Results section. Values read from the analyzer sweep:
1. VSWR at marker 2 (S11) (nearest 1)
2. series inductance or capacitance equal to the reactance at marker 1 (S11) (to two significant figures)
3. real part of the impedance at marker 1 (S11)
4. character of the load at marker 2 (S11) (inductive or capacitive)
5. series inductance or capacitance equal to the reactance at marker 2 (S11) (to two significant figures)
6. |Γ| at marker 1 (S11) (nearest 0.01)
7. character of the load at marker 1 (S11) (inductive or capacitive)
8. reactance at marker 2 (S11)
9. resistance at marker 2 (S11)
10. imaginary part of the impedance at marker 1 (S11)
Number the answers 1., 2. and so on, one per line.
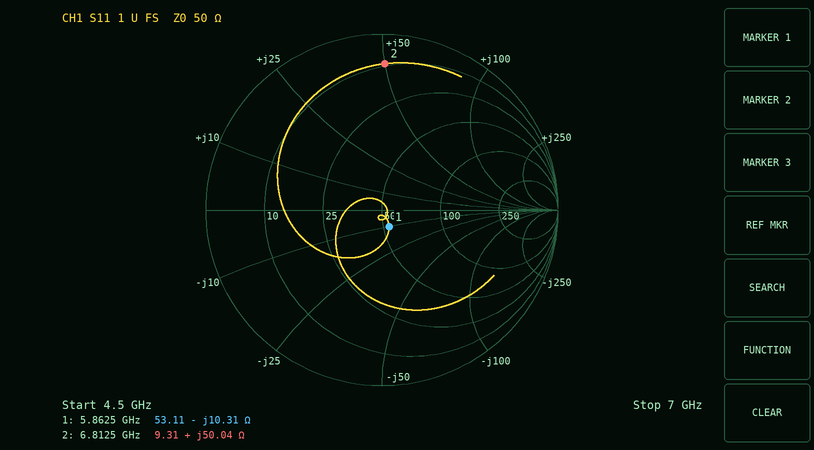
1. 11
2. 2.6 pF
3. 53.11 Ω
4. inductive
5. 1.2 nH
6. 0.10
7. capacitive
8. +50.04 Ω
9. 9.31 Ω
10. -10.31 Ω
